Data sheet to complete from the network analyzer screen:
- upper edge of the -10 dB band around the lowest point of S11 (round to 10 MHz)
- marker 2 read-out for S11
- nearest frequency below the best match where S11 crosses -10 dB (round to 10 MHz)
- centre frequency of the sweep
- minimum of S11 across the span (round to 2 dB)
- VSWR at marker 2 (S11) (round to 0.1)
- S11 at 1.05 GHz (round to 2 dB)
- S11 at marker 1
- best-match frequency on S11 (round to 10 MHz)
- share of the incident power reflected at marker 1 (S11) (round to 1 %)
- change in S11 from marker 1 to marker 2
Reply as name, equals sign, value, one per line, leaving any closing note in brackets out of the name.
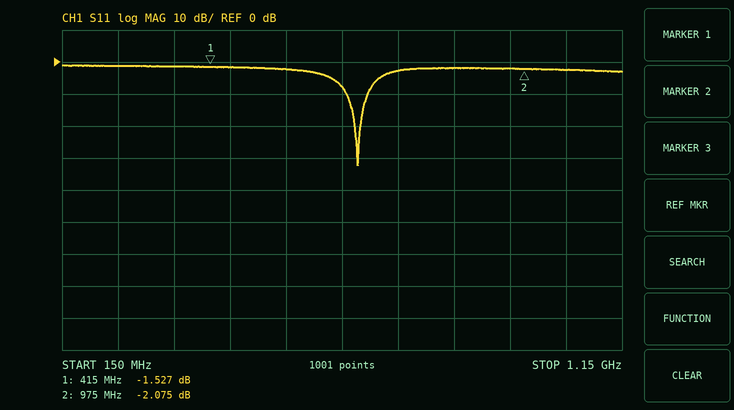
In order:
upper edge of the -10 dB band around the lowest point of S11 = 700 MHz
marker 2 read-out for S11 = -2.075 dB
nearest frequency below the best match where S11 crosses -10 dB = 660 MHz
centre frequency of the sweep = 650 MHz
minimum of S11 across the span = -32 dB
VSWR at marker 2 (S11) = 8.4
S11 at 1.05 GHz = -2 dB
S11 at marker 1 = -1.527 dB
best-match frequency on S11 = 680 MHz
share of the incident power reflected at marker 1 (S11) = 70 %
change in S11 from marker 1 to marker 2 = -0.548 dB
